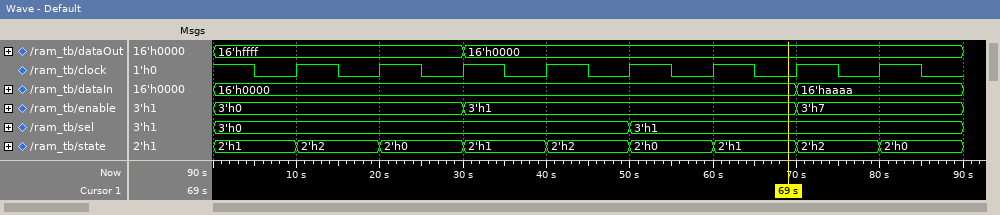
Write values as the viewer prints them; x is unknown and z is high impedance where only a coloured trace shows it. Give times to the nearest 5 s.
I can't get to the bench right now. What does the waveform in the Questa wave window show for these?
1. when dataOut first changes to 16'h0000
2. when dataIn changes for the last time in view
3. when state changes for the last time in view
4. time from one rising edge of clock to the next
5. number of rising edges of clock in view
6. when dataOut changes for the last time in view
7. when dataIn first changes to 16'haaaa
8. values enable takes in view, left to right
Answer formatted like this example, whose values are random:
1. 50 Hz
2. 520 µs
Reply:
1. 30 s
2. 70 s
3. 80 s
4. 10 s
5. 8
6. 30 s
7. 70 s
8. 3'h0, 3'h1, 3'h7
